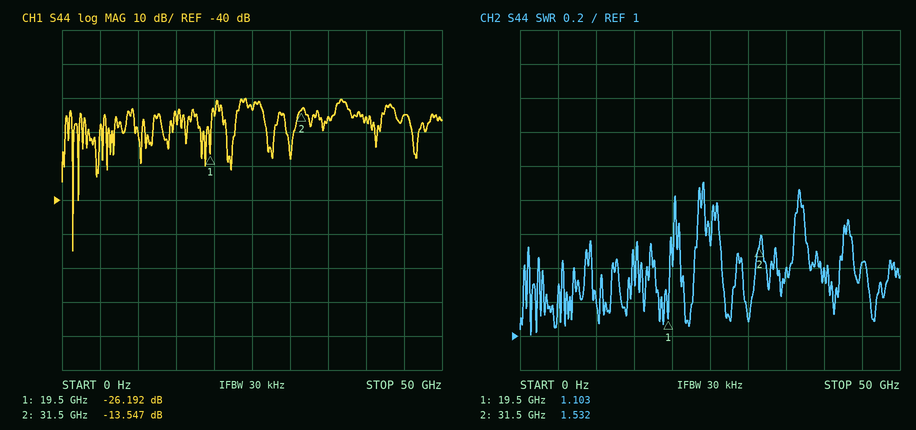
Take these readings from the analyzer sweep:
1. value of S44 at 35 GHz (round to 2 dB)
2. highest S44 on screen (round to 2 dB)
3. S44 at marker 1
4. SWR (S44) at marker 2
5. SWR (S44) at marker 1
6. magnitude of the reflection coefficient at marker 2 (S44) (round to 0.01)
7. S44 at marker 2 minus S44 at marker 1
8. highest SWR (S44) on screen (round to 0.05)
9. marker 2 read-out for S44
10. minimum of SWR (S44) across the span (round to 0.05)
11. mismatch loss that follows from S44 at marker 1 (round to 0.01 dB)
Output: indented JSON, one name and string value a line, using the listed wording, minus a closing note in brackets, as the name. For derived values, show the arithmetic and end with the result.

{
  "value of S44 at 35 GHz": "-16 dB",
  "highest S44 on screen": "-10 dB",
  "S44 at marker 1": "-26.192 dB",
  "SWR (S44) at marker 2": "1.532",
  "SWR (S44) at marker 1": "1.103",
  "magnitude of the reflection coefficient at marker 2 (S44)": "10^(-13.547/20) ≈ 0.21",
  "S44 at marker 2 minus S44 at marker 1": "-13.547 − (-26.192) = 12.645 dB",
  "highest SWR (S44) on screen": "1.90",
  "marker 2 read-out for S44": "-13.547 dB",
  "minimum of SWR (S44) across the span": "1.00",
  "mismatch loss that follows from S44 at marker 1": "−10 log10(1 − 10^(-26.192/10)) ≈ 0.01 dB"
}
